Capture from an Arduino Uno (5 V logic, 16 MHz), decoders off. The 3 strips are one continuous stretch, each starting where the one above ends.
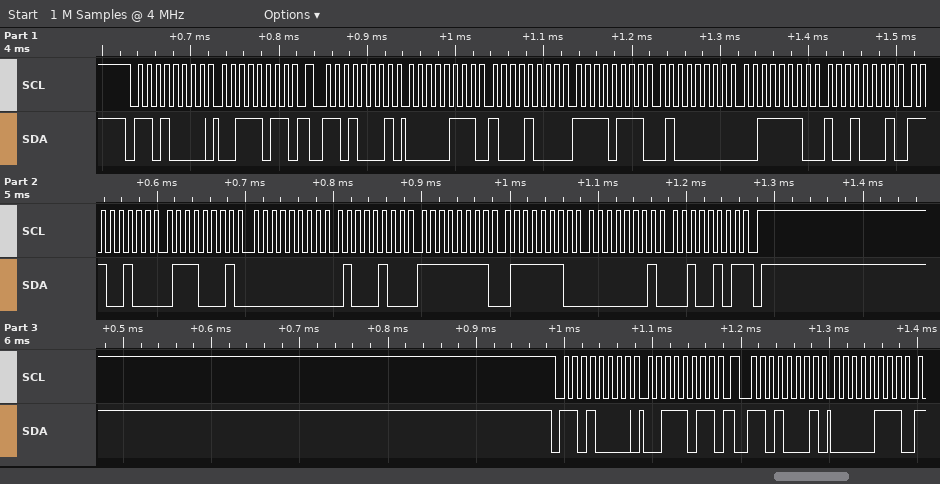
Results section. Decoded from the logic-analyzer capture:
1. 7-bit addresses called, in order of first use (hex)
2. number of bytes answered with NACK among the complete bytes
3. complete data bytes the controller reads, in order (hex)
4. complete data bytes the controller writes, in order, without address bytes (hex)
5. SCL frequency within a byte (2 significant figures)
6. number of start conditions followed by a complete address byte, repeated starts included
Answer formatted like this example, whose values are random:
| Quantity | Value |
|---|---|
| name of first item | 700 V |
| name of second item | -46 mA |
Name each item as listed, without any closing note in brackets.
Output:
| Quantity | Value |
|---|---|
| 7-bit addresses called, in order of first use | 0x68 |
| number of bytes answered with NACK among the complete bytes | 1 |
| complete data bytes the controller reads, in order | 07 88 F7 40 3E 91 E4 71 00 44 FF 7E 01 25 07 |
| complete data bytes the controller writes, in order, without address bytes | 3B 3B |
| SCL frequency within a byte | 100 kHz |
| number of start conditions followed by a complete address byte, repeated starts included | 4 |
